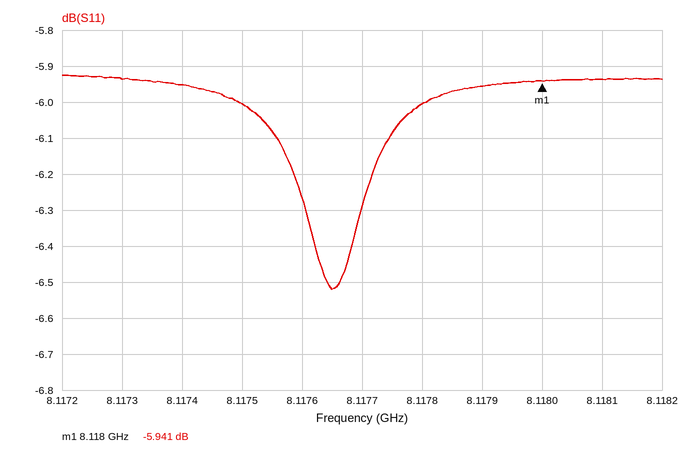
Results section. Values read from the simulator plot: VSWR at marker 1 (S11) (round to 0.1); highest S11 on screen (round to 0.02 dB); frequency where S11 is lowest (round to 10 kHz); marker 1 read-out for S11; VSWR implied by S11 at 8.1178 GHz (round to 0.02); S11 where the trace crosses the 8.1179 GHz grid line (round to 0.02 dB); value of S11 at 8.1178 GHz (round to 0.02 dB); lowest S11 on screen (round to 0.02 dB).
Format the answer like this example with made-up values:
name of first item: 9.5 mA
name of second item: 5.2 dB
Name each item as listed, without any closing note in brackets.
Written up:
VSWR at marker 1 (S11): 3.0
highest S11 on screen: -5.92 dB
frequency where S11 is lowest: 8.11765 GHz
marker 1 read-out for S11: -5.941 dB
VSWR implied by S11 at 8.1178 GHz: 3.00
S11 where the trace crosses the 8.1179 GHz grid line: -5.96 dB
value of S11 at 8.1178 GHz: -6.00 dB
lowest S11 on screen: -6.52 dB
